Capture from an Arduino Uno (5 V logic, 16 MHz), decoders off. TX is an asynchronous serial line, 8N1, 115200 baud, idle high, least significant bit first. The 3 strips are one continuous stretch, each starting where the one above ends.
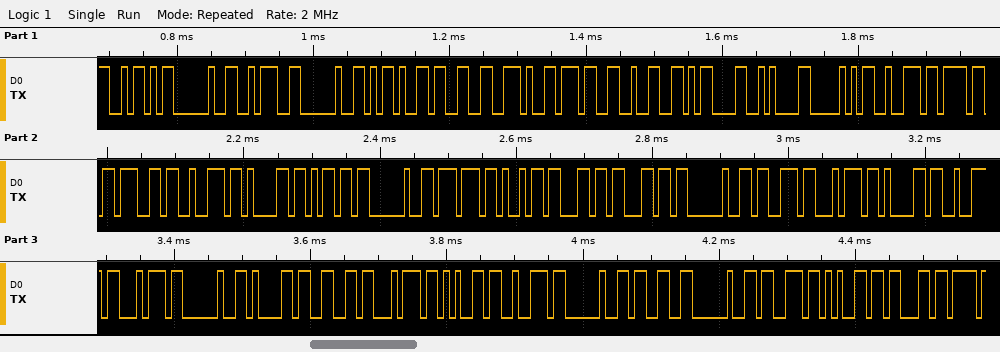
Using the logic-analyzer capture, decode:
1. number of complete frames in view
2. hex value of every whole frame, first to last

41
0x5A 0x20 0x3A 0x20 0x2D 0x33 0x2E 0x37 0x32 0x0D 0x0A 0x50 0x72 0x6F 0x67 0x72 0x61 0x6D 0x20 0x77 0x69 0x6C 0x6C 0x20 0x73 0x74 0x61 0x72 0x74 0x20 0x61 0x66 0x74 0x65 0x72 0x20 0x33 0x20 0x73 0x65 0x63
